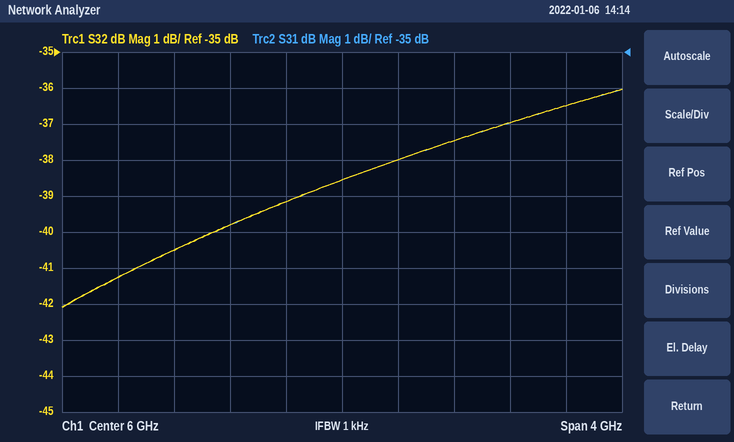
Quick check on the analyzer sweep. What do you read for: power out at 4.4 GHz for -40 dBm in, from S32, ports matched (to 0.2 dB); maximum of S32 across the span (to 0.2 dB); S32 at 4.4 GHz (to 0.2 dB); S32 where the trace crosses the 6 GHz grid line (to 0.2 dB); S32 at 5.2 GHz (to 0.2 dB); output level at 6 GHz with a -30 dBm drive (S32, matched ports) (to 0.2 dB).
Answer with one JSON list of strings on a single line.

["-81.2 dBm", "-36.0 dB", "-41.2 dB", "-38.6 dB", "-39.8 dB", "-68.6 dBm"]
